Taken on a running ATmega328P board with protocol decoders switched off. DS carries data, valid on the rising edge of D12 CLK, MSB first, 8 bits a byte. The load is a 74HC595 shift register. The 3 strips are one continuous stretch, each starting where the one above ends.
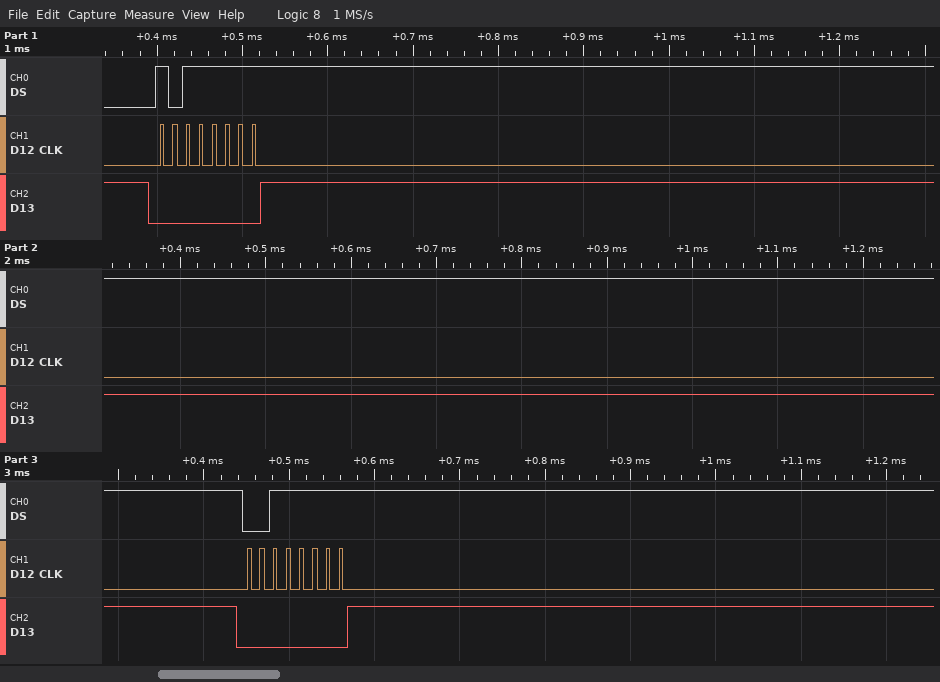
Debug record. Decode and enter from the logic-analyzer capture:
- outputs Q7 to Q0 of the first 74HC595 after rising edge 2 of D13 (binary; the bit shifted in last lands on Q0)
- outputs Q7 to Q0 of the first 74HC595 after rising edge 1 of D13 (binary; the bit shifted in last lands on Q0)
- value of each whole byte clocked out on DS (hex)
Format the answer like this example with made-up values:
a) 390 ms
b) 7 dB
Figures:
a) 00111111
b) 10111111
c) BF 3F
